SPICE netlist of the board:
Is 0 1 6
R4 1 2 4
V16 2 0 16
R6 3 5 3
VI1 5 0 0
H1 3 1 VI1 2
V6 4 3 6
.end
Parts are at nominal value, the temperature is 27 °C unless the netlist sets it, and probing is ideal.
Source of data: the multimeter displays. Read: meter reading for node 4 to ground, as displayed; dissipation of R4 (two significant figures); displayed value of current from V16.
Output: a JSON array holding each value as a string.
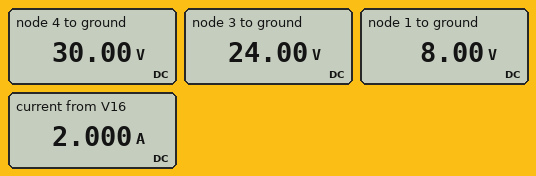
["30.00 V", "16 W", "2.000 A"]
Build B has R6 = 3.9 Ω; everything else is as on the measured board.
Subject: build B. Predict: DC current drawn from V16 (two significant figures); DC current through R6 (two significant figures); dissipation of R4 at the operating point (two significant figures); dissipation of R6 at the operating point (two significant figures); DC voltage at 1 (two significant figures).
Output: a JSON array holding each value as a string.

["780 mA", "6.8 A", "2.4 W", "180 W", "13 V"]
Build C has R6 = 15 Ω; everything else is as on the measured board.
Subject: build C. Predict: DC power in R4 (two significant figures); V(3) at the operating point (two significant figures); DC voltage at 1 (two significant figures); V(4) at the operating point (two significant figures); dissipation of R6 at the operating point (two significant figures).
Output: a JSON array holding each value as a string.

["53 W", "35 V", "31 V", "41 V", "83 W"]
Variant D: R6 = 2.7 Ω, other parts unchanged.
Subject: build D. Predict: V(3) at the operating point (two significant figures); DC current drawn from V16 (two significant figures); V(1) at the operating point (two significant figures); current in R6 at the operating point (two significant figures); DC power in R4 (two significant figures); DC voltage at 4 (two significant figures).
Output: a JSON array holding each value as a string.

["23 V", "2.5 A", "6.0 V", "8.5 A", "25 W", "29 V"]
